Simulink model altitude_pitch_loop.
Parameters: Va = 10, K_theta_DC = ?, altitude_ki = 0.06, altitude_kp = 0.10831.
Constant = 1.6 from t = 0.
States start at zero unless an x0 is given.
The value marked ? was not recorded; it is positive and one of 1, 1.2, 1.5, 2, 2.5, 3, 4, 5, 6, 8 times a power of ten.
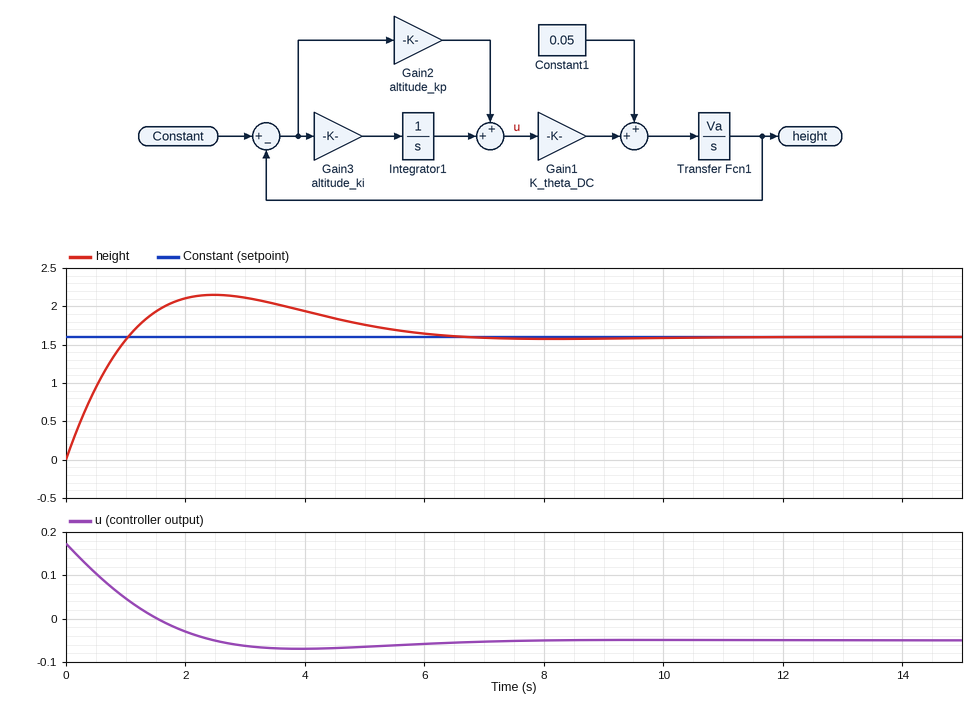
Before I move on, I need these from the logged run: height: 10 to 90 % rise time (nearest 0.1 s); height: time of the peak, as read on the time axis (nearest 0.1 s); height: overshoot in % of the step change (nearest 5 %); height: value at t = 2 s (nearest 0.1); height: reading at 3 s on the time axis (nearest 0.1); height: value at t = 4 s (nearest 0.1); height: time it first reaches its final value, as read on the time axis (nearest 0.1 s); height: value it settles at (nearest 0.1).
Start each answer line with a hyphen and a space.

- 0.8 s
- 2.5 s
- 35 %
- 2.1
- 2.1
- 1.9
- 1.0 s
- 1.6
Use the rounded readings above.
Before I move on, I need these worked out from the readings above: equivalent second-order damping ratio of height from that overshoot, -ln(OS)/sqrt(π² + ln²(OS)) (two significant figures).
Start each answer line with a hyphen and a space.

- 0.32
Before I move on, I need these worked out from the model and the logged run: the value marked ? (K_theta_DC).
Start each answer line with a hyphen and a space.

- 1
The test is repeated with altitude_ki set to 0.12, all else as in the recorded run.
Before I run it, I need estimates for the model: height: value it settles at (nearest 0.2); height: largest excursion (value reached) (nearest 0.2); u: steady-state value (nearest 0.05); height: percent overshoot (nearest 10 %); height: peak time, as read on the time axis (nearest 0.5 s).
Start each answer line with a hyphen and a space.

- 1.6
- 2.2
- -0.05
- 40 %
- 2.0 s
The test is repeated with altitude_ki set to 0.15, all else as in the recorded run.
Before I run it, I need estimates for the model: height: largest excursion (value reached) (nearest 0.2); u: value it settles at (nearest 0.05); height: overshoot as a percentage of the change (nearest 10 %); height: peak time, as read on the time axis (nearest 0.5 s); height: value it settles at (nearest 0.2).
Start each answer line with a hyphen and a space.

- 2.2
- -0.05
- 40 %
- 2.0 s
- 1.6
